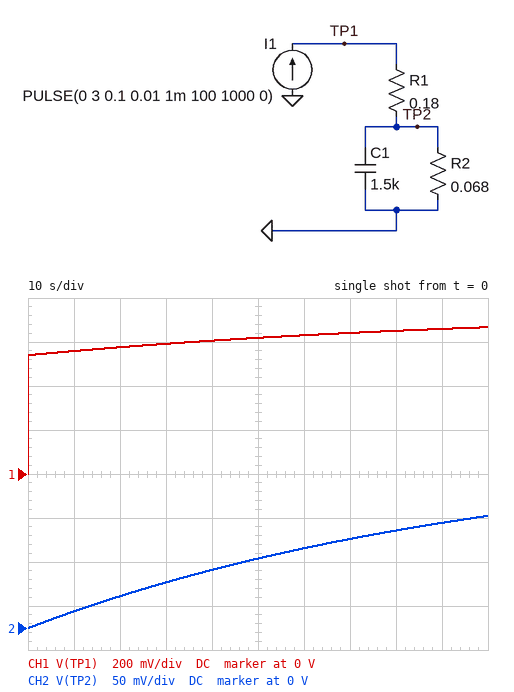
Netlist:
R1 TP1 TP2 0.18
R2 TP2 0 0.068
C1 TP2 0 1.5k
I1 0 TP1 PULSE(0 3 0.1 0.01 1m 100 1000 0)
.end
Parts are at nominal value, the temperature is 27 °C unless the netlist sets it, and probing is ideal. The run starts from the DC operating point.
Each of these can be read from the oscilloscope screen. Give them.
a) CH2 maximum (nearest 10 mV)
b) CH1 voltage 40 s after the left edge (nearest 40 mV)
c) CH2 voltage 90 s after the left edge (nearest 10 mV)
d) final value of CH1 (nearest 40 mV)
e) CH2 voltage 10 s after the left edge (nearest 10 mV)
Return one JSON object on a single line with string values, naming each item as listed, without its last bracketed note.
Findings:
{"CH2 maximum": "130 mV", "CH1 voltage 40 s after the left edge": "600 mV", "CH2 voltage 90 s after the left edge": "120 mV", "final value of CH1": "680 mV", "CH2 voltage 10 s after the left edge": "20 mV"}
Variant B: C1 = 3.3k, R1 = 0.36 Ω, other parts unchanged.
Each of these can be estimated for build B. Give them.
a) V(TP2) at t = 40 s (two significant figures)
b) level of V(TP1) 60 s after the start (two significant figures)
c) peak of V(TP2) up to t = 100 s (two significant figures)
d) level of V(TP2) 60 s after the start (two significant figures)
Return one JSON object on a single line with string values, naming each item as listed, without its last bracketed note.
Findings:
{"V(TP2) at t = 40 s": "33 mV", "level of V(TP1) 60 s after the start": "1.1 V", "peak of V(TP2) up to t = 100 s": "73 mV", "level of V(TP2) 60 s after the start": "48 mV"}
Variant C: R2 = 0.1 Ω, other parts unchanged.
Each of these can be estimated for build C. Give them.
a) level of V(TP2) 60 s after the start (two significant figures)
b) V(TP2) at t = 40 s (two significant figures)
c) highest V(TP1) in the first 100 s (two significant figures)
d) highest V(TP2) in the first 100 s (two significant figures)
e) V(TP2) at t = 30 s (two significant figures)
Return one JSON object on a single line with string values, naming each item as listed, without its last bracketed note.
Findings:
{"level of V(TP2) 60 s after the start": "99 mV", "V(TP2) at t = 40 s": "70 mV", "highest V(TP1) in the first 100 s": "690 mV", "highest V(TP2) in the first 100 s": "150 mV", "V(TP2) at t = 30 s": "54 mV"}
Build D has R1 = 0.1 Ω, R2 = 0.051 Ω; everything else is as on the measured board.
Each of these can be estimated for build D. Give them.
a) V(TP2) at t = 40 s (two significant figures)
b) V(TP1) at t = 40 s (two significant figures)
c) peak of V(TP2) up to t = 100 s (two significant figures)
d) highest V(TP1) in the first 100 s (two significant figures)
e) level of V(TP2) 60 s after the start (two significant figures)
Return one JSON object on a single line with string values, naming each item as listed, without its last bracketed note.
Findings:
{"V(TP2) at t = 40 s": "62 mV", "V(TP1) at t = 40 s": "360 mV", "peak of V(TP2) up to t = 100 s": "110 mV", "highest V(TP1) in the first 100 s": "410 mV", "level of V(TP2) 60 s after the start": "83 mV"}
